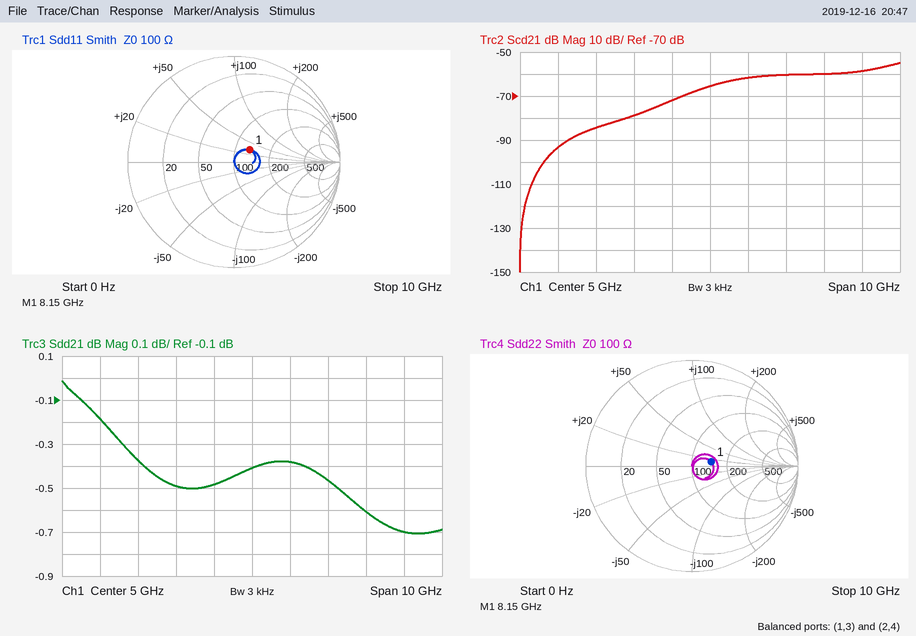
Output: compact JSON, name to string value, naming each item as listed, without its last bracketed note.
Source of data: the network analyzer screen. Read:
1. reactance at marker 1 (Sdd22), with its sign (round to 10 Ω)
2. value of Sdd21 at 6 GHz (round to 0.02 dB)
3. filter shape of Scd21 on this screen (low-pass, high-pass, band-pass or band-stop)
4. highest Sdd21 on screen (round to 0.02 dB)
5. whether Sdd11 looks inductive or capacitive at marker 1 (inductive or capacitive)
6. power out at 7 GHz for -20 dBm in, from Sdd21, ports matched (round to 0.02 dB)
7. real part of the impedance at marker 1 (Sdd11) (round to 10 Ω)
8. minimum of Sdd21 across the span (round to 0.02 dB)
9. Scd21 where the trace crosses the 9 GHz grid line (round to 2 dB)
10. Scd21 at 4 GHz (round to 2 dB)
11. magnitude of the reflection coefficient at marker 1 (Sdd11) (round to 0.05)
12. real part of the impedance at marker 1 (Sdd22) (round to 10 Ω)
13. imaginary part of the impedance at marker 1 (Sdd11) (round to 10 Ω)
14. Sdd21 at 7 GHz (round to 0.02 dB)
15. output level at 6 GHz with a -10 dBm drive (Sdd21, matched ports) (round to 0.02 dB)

{"reactance at marker 1 (Sdd22), with its sign": "+10 Ω", "value of Sdd21 at 6 GHz": "-0.38 dB", "filter shape of Scd21 on this screen": "high-pass", "highest Sdd21 on screen": "-0.02 dB", "whether Sdd11 looks inductive or capacitive at marker 1": "inductive", "power out at 7 GHz for -20 dBm in, from Sdd21, ports matched": "-20.46 dBm", "real part of the impedance at marker 1 (Sdd11)": "130 Ω", "minimum of Sdd21 across the span": "-0.70 dB", "Scd21 where the trace crosses the 9 GHz grid line": "-58 dB", "Scd21 at 4 GHz": "-72 dB", "magnitude of the reflection coefficient at marker 1 (Sdd11)": "0.20", "real part of the impedance at marker 1 (Sdd22)": "140 Ω", "imaginary part of the impedance at marker 1 (Sdd11)": "+30 Ω", "Sdd21 at 7 GHz": "-0.46 dB", "output level at 6 GHz with a -10 dBm drive (Sdd21, matched ports)": "-10.38 dBm"}
